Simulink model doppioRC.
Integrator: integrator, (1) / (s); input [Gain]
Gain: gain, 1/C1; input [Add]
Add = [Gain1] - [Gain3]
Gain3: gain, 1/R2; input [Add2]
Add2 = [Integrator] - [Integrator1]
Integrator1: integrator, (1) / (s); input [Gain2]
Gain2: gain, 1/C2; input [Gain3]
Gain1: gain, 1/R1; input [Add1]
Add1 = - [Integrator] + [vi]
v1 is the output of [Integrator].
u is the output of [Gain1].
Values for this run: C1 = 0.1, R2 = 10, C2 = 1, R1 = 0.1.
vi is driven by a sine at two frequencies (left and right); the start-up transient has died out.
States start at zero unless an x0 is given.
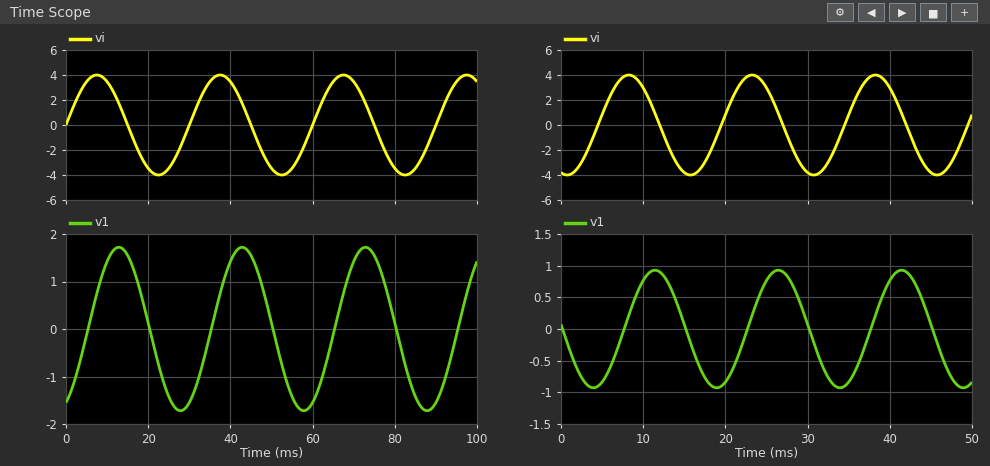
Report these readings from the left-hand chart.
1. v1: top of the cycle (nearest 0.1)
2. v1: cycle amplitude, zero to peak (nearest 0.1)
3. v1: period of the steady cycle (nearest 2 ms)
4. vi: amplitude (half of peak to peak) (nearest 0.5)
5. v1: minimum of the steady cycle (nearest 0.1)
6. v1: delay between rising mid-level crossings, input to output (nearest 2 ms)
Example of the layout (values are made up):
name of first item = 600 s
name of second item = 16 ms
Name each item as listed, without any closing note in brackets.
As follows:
v1: top of the cycle = 1.7
v1: cycle amplitude, zero to peak = 1.7
v1: period of the steady cycle = 30 ms
vi: amplitude (half of peak to peak) = 4.0
v1: minimum of the steady cycle = -1.7
v1: delay between rising mid-level crossings, input to output = 6 ms
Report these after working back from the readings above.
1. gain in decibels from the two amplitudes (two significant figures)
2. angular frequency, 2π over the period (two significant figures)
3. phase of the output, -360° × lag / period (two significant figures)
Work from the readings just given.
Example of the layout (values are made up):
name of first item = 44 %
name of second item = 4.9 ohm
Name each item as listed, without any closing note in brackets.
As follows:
gain in decibels from the two amplitudes = -7.4 dB
angular frequency, 2π over the period = 0.21 rad/ms
phase of the output, -360° × lag / period = -72°
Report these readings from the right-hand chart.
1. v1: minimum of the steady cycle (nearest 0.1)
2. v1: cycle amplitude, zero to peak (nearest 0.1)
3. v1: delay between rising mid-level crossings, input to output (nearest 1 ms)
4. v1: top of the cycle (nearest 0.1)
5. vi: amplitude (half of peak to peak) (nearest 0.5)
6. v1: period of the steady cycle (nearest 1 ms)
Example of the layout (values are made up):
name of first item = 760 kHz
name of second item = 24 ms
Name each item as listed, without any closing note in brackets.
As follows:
v1: minimum of the steady cycle = -0.9
v1: cycle amplitude, zero to peak = 0.9
v1: delay between rising mid-level crossings, input to output = 3 ms
v1: top of the cycle = 0.9
vi: amplitude (half of peak to peak) = 4.0
v1: period of the steady cycle = 15 ms
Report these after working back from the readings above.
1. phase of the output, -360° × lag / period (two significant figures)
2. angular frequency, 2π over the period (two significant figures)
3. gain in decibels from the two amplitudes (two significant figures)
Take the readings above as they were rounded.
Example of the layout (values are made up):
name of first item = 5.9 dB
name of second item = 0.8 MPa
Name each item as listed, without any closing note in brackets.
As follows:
phase of the output, -360° × lag / period = -72°
angular frequency, 2π over the period = 0.42 rad/ms
gain in decibels from the two amplitudes = -13 dB
